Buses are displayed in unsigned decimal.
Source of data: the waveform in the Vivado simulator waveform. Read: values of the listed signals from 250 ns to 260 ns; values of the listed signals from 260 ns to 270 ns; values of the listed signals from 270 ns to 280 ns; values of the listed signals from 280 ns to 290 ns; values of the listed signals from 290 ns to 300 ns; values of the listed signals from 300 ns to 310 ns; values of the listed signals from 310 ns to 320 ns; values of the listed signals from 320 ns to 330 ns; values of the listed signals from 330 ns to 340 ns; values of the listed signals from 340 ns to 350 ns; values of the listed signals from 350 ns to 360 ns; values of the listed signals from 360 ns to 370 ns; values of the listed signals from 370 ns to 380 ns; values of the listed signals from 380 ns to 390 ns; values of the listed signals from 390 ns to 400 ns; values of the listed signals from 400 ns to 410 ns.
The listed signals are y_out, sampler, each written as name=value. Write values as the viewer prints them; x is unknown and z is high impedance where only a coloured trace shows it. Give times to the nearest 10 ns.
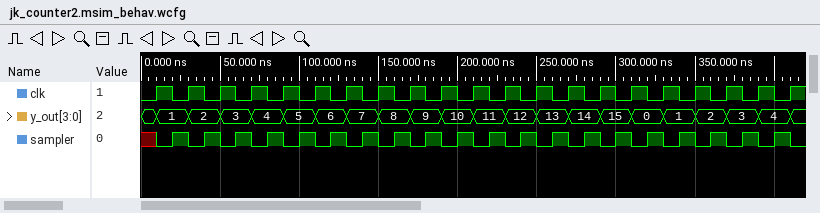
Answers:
y_out=13, sampler=0
y_out=13, sampler=1
y_out=14, sampler=0
y_out=14, sampler=1
y_out=15, sampler=0
y_out=15, sampler=1
y_out=0, sampler=0
y_out=0, sampler=1
y_out=1, sampler=0
y_out=1, sampler=1
y_out=2, sampler=0
y_out=2, sampler=1
y_out=3, sampler=0
y_out=3, sampler=1
y_out=4, sampler=0
y_out=4, sampler=1
